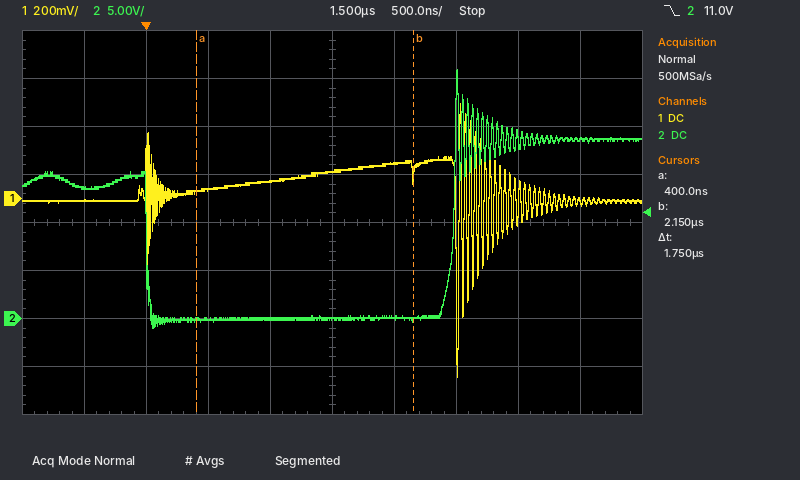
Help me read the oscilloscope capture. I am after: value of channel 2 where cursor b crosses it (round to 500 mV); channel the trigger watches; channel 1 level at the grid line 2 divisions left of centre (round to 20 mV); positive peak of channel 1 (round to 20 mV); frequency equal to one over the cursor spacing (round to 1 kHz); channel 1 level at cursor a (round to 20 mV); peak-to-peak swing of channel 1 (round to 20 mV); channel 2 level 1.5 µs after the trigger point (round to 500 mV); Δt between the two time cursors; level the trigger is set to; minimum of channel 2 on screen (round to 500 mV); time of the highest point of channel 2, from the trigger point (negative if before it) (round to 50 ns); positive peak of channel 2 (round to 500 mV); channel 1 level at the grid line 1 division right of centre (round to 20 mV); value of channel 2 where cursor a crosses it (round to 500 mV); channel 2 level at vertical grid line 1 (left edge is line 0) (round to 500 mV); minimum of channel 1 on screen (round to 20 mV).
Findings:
0.0 V
channel 2
40 mV
400 mV
571 kHz
20 mV
1.14 V
0.0 V
1.75 µs
11.0 V
-1.0 V
+2.50 µs
26.0 V
140 mV
0.0 V
13.5 V
-740 mV
